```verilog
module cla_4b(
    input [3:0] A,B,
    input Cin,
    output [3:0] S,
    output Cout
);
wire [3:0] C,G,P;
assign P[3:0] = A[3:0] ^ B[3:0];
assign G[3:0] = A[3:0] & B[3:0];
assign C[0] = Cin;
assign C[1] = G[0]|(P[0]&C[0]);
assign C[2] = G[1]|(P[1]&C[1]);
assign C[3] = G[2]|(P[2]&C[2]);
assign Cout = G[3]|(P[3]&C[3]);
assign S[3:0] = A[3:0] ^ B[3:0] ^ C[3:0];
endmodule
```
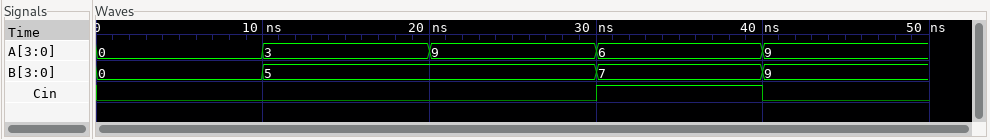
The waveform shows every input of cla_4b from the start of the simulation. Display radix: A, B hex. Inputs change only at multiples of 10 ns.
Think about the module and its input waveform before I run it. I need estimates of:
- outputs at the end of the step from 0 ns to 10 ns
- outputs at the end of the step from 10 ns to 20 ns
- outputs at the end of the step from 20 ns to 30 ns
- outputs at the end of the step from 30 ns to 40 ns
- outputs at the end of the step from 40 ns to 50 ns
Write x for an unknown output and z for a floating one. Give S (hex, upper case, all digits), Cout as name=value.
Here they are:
S=0, Cout=0
S=8, Cout=0
S=E, Cout=0
S=E, Cout=0
S=2, Cout=1
